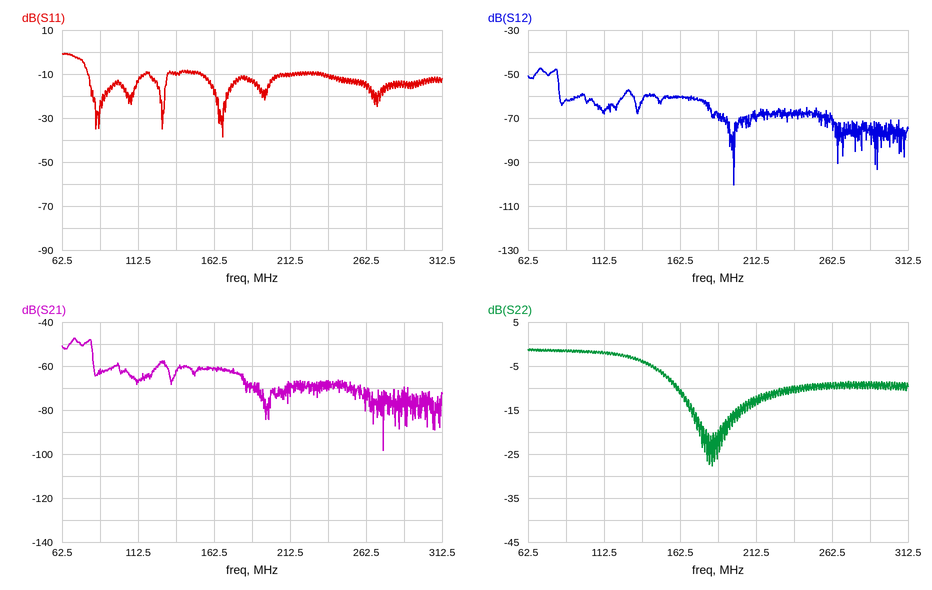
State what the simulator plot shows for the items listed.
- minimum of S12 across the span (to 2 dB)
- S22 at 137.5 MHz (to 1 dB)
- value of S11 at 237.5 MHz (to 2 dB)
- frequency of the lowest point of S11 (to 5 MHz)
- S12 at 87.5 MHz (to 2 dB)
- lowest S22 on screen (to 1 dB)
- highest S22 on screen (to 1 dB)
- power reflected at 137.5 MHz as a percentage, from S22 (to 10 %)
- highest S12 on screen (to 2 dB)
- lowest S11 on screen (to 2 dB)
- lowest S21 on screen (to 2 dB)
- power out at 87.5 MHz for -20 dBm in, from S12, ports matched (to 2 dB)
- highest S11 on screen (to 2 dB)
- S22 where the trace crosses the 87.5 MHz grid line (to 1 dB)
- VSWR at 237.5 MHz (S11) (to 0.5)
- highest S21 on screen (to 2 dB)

-100 dB
-4 dB
-10 dB
170 MHz
-62 dB
-28 dB
-1 dB
40 %
-48 dB
-38 dB
-98 dB
-82 dBm
0 dB
-1 dB
2.0
-48 dB
